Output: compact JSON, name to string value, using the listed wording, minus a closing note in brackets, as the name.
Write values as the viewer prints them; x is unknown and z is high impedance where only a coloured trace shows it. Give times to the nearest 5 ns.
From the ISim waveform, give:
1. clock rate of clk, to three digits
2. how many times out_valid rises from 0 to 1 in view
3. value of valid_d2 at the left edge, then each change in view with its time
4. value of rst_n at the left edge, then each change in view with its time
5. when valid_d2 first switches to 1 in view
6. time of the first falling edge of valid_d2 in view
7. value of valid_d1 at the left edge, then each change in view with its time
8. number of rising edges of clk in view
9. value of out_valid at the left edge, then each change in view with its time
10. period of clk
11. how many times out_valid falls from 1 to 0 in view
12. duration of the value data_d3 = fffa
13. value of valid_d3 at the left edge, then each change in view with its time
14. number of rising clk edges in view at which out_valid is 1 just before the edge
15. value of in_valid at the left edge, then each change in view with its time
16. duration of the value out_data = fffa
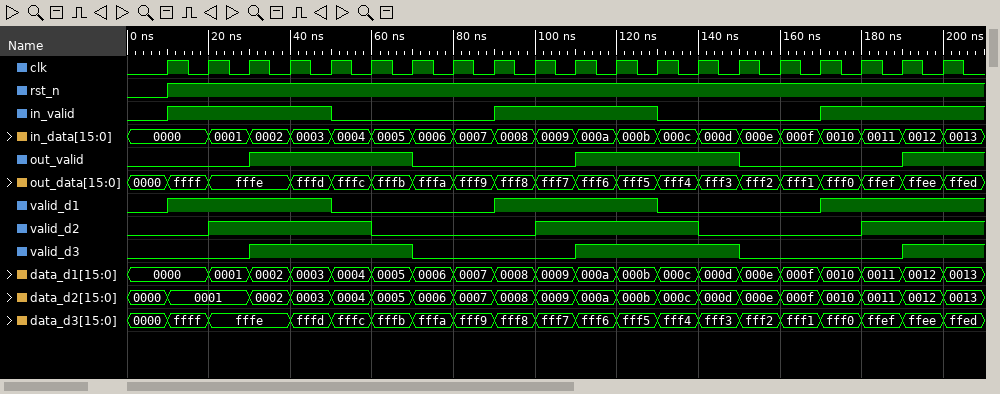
{"clock rate of clk, to three digits": "100 MHz", "how many times out_valid rises from 0 to 1 in view": "3", "value of valid_d2 at the left edge, then each change in view with its time": "0, 1 at 20 ns, 0 at 60 ns, 1 at 100 ns, 0 at 140 ns, 1 at 180 ns", "value of rst_n at the left edge, then each change in view with its time": "0, 1 at 10 ns", "when valid_d2 first switches to 1 in view": "20 ns", "time of the first falling edge of valid_d2 in view": "60 ns", "value of valid_d1 at the left edge, then each change in view with its time": "0, 1 at 10 ns, 0 at 50 ns, 1 at 90 ns, 0 at 130 ns, 1 at 170 ns", "number of rising edges of clk in view": "20", "value of out_valid at the left edge, then each change in view with its time": "0, 1 at 30 ns, 0 at 70 ns, 1 at 110 ns, 0 at 150 ns, 1 at 190 ns", "period of clk": "10 ns", "how many times out_valid falls from 1 to 0 in view": "2", "duration of the value data_d3 = fffa": "10 ns", "value of valid_d3 at the left edge, then each change in view with its time": "0, 1 at 30 ns, 0 at 70 ns, 1 at 110 ns, 0 at 150 ns, 1 at 190 ns", "number of rising clk edges in view at which out_valid is 1 just before the edge": "9", "value of in_valid at the left edge, then each change in view with its time": "0, 1 at 10 ns, 0 at 50 ns, 1 at 90 ns, 0 at 130 ns, 1 at 170 ns", "duration of the value out_data = fffa": "10 ns"}
